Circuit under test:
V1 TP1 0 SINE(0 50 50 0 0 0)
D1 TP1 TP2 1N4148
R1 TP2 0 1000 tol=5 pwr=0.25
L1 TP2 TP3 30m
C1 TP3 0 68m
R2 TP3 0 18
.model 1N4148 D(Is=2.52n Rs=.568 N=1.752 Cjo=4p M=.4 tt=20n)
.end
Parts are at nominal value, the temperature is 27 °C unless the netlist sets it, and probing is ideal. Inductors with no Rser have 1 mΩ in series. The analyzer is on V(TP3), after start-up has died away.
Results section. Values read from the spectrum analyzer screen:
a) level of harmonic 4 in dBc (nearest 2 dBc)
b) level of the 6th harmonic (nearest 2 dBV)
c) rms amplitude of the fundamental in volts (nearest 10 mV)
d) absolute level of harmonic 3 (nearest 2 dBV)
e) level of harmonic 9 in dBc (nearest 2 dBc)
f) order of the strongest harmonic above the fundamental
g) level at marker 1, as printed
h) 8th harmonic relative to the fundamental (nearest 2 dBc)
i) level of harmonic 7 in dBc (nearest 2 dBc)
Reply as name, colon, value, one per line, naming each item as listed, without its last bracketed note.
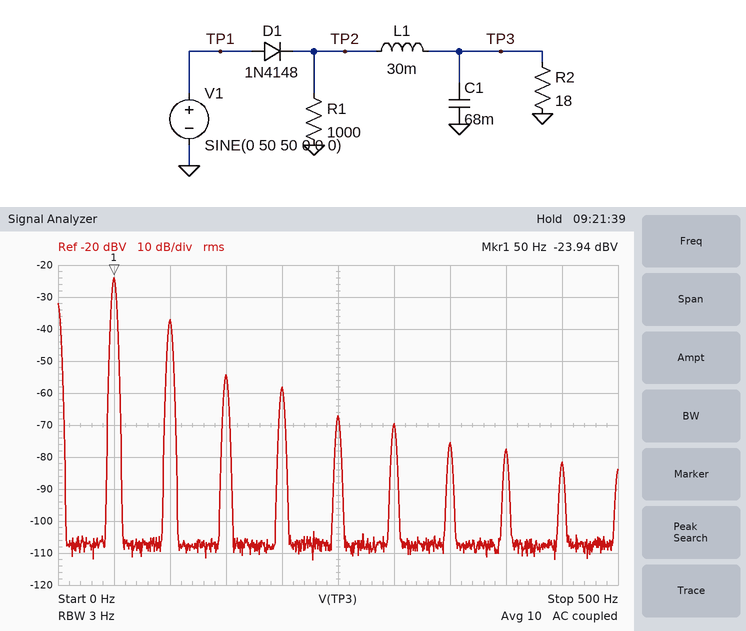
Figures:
level of harmonic 4 in dBc: -34 dBc
level of the 6th harmonic: -70 dBV
rms amplitude of the fundamental in volts: 60 mV
absolute level of harmonic 3: -54 dBV
level of harmonic 9 in dBc: -58 dBc
order of the strongest harmonic above the fundamental: 2
level at marker 1, as printed: -23.94 dBV
8th harmonic relative to the fundamental: -54 dBc
level of harmonic 7 in dBc: -52 dBc
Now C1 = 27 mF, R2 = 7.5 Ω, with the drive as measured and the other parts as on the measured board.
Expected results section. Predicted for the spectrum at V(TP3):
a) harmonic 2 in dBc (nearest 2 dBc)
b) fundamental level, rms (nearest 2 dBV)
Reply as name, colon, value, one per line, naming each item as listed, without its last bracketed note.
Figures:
harmonic 2 in dBc: -16 dBc
fundamental level, rms: -12 dBV
